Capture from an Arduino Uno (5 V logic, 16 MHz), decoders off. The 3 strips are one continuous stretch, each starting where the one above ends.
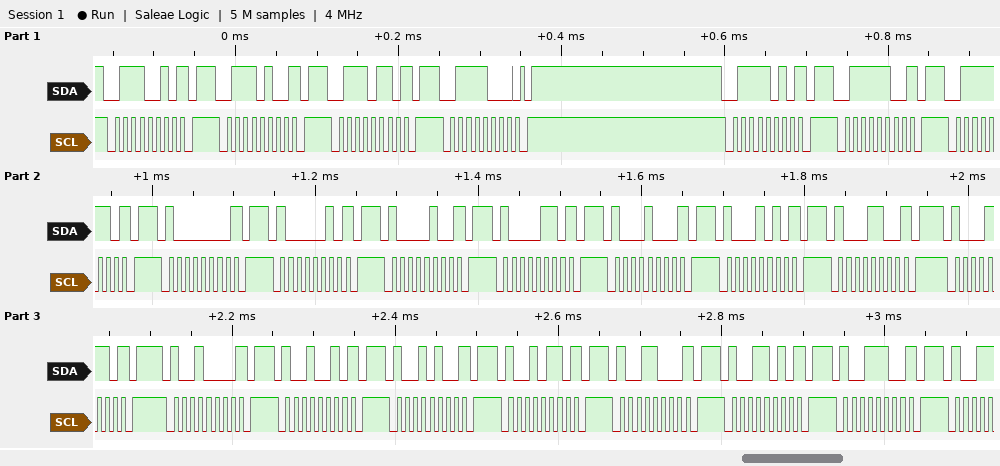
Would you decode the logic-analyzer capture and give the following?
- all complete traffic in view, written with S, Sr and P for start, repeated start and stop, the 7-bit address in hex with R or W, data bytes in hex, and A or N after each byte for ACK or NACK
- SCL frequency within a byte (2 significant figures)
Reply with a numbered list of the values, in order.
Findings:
1. S 39W N P S 3AW N P S 3BW N P S 3CW A P S 3DW N P S 3EW N P S 3FW N P S 40W N P S 41W N P S 42W N P S 43W N P S 44W N P S 45W N P S 46W N P S 47W N P S 48W N P S 49W N P S 4AW N P S 4BW N P S 4CW N P S 4DW N P S 4EW N P
2. 100 kHz
